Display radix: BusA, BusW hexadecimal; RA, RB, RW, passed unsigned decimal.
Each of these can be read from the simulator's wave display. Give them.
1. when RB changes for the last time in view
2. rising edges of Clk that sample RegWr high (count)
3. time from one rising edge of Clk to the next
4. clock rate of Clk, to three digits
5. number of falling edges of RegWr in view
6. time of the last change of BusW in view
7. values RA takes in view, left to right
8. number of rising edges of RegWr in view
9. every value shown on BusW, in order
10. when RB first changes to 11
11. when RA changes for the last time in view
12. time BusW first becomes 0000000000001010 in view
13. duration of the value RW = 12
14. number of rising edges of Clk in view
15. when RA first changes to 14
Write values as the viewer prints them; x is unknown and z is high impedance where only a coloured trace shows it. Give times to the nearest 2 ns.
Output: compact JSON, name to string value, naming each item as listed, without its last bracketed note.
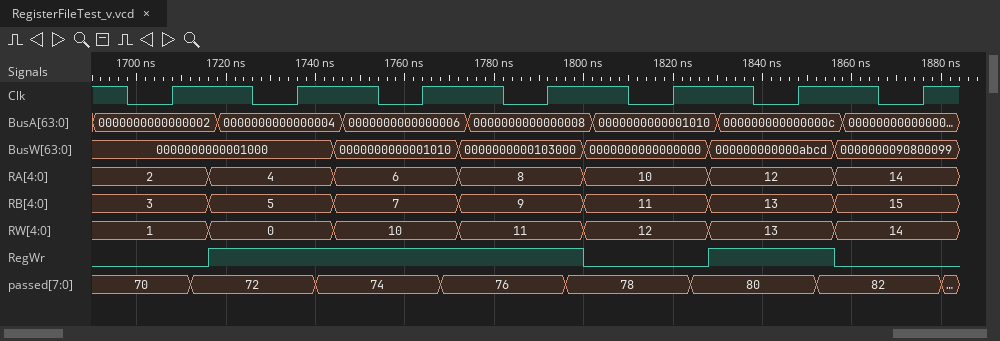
{"when RB changes for the last time in view": "1856 ns", "rising edges of Clk that sample RegWr high": "4", "time from one rising edge of Clk to the next": "28 ns", "clock rate of Clk, to three digits": "35.7 MHz", "number of falling edges of RegWr in view": "2", "time of the last change of BusW in view": "1856 ns", "values RA takes in view, left to right": "2, 4, 6, 8, 10, 12, 14", "number of rising edges of RegWr in view": "2", "every value shown on BusW, in order": "0000000000001000, 0000000000001010, 0000000000103000, 0000000000000000, 000000000000abcd, 0000000090800099", "when RB first changes to 11": "1800 ns", "when RA changes for the last time in view": "1856 ns", "time BusW first becomes 0000000000001010 in view": "1744 ns", "duration of the value RW = 12": "28 ns", "number of rising edges of Clk in view": "7", "when RA first changes to 14": "1856 ns"}
